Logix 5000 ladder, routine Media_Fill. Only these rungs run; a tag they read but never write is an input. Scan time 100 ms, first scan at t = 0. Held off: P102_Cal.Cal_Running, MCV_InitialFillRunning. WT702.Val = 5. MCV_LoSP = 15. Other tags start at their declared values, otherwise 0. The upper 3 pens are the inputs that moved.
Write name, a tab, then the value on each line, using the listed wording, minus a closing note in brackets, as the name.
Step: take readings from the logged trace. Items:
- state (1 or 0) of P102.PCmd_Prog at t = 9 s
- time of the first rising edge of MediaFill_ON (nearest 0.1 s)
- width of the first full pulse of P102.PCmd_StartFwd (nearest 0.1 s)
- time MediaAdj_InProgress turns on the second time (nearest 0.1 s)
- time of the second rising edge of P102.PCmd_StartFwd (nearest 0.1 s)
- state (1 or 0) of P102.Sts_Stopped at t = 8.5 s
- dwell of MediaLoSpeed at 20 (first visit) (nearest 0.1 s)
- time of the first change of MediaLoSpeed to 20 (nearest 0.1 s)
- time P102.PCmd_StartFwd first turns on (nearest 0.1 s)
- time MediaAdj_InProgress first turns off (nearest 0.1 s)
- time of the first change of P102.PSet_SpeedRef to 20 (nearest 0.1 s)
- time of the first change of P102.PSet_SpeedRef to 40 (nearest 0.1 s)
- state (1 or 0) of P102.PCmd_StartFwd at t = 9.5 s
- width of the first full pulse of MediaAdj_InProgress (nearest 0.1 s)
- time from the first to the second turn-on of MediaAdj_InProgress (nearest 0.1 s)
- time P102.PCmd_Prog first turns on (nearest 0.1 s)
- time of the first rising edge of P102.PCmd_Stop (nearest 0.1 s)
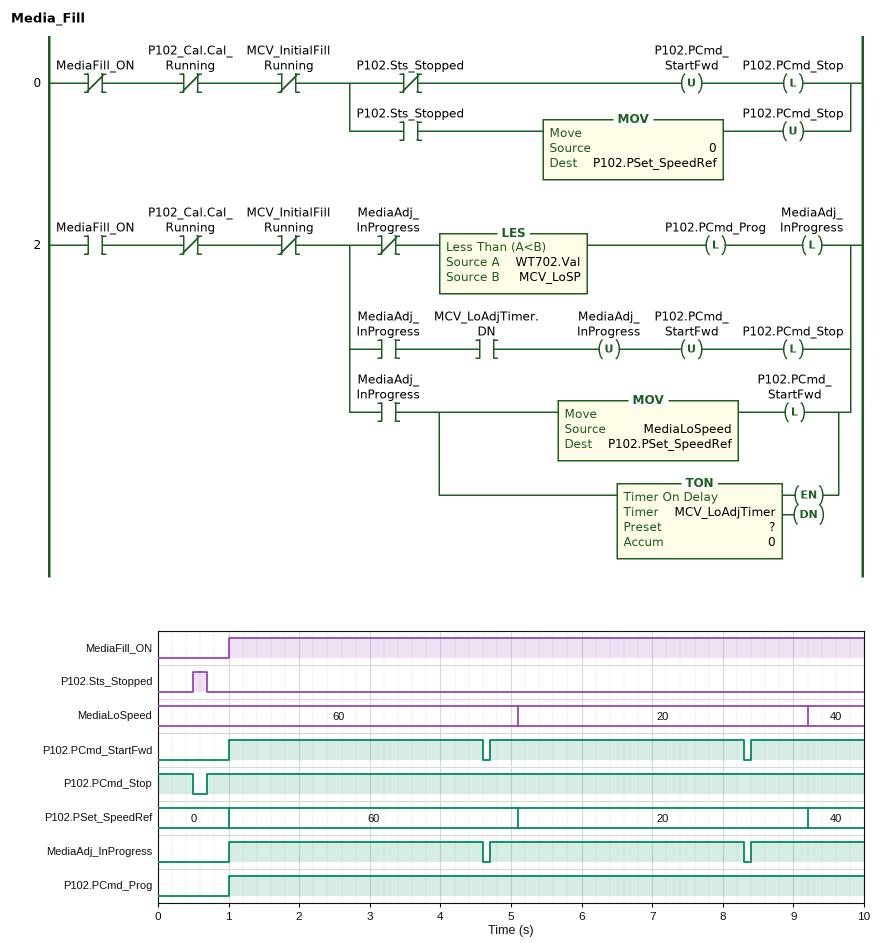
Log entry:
state (1 or 0) of P102.PCmd_Prog at t = 9 s	1
time of the first rising edge of MediaFill_ON	1.0 s
width of the first full pulse of P102.PCmd_StartFwd	3.6 s
time MediaAdj_InProgress turns on the second time	4.7 s
time of the second rising edge of P102.PCmd_StartFwd	4.7 s
state (1 or 0) of P102.Sts_Stopped at t = 8.5 s	0
dwell of MediaLoSpeed at 20 (first visit)	4.1 s
time of the first change of MediaLoSpeed to 20	5.1 s
time P102.PCmd_StartFwd first turns on	1.0 s
time MediaAdj_InProgress first turns off	4.6 s
time of the first change of P102.PSet_SpeedRef to 20	5.1 s
time of the first change of P102.PSet_SpeedRef to 40	9.2 s
state (1 or 0) of P102.PCmd_StartFwd at t = 9.5 s	1
width of the first full pulse of MediaAdj_InProgress	3.6 s
time from the first to the second turn-on of MediaAdj_InProgress	3.7 s
time P102.PCmd_Prog first turns on	1.0 s
time of the first rising edge of P102.PCmd_Stop	0.7 s
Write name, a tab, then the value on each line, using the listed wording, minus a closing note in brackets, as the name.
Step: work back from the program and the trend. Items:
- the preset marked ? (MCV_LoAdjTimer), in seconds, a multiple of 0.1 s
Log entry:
the preset marked ? (MCV_LoAdjTimer), in seconds, a multiple of 0.1 s	3.5 s
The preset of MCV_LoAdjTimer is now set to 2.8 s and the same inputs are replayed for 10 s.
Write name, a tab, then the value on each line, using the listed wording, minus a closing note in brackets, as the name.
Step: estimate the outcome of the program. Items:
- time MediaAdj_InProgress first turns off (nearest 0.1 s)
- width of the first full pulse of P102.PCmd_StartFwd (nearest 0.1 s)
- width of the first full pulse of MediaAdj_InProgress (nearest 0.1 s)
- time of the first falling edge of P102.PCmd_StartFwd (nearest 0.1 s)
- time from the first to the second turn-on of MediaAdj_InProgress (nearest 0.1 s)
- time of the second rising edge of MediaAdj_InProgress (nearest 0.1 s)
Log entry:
time MediaAdj_InProgress first turns off	3.9 s
width of the first full pulse of P102.PCmd_StartFwd	2.9 s
width of the first full pulse of MediaAdj_InProgress	2.9 s
time of the first falling edge of P102.PCmd_StartFwd	3.9 s
time from the first to the second turn-on of MediaAdj_InProgress	3.0 s
time of the second rising edge of MediaAdj_InProgress	4.0 s
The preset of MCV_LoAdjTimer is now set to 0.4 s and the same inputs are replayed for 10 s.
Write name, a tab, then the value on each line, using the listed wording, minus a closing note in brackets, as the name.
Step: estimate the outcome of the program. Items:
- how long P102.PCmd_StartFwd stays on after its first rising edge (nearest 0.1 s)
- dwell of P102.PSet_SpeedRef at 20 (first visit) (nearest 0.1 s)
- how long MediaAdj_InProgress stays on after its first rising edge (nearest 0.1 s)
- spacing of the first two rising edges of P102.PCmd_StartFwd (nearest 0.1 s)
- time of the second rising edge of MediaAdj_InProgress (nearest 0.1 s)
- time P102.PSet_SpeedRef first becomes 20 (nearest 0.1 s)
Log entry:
how long P102.PCmd_StartFwd stays on after its first rising edge	0.5 s
dwell of P102.PSet_SpeedRef at 20 (first visit)	4.0 s
how long MediaAdj_InProgress stays on after its first rising edge	0.5 s
spacing of the first two rising edges of P102.PCmd_StartFwd	0.6 s
time of the second rising edge of MediaAdj_InProgress	1.6 s
time P102.PSet_SpeedRef first becomes 20	5.2 s
